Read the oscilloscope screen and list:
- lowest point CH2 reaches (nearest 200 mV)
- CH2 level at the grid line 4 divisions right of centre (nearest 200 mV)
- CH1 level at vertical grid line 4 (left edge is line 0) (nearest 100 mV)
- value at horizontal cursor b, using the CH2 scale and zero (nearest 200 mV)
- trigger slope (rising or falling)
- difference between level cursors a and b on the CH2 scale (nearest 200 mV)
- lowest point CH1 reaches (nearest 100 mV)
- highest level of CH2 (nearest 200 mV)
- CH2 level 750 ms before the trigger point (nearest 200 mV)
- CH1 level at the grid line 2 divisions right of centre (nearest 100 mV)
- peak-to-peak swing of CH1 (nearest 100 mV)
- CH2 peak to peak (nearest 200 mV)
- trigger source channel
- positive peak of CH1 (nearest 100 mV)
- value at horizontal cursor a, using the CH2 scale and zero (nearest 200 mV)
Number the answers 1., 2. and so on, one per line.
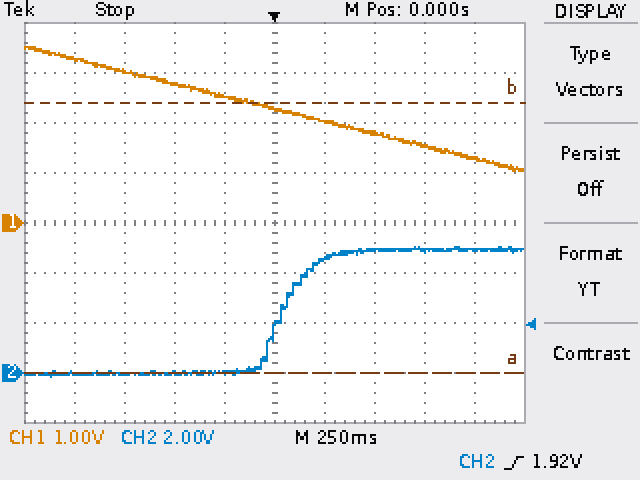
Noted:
1. -200 mV
2. 5.0 V
3. 2.5 V
4. 10.8 V
5. rising
6. 10.8 V
7. 1.0 V
8. 5.0 V
9. 0.0 V
10. 1.8 V
11. 2.5 V
12. 5.2 V
13. CH2
14. 3.5 V
15. 0.0 V
